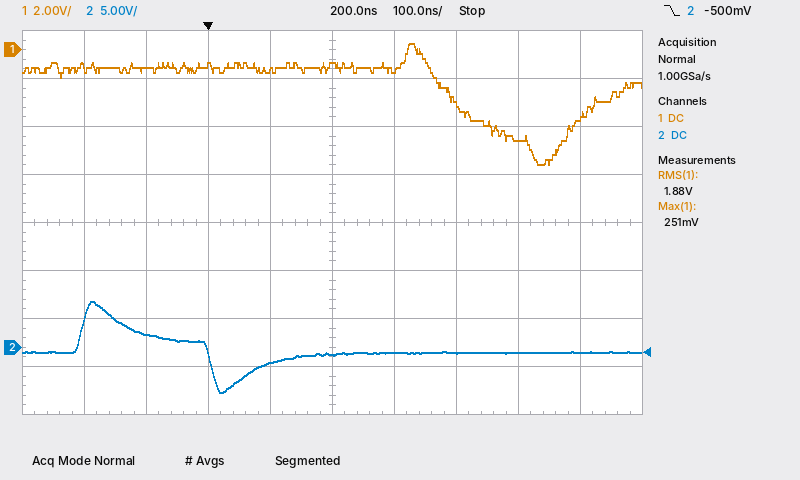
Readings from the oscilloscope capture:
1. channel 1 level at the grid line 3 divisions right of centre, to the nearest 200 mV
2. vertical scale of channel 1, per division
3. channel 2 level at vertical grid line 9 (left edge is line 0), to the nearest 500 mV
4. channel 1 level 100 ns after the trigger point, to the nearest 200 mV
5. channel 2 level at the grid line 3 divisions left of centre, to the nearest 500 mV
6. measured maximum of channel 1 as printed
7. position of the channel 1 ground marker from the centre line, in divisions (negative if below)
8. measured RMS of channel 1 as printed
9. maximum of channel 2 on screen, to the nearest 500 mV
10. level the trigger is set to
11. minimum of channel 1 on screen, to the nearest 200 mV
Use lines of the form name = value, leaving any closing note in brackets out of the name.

channel 1 level at the grid line 3 divisions right of centre, to the nearest 200 mV = -3.8 V
vertical scale of channel 1, per division = 2 V
channel 2 level at vertical grid line 9 (left edge is line 0), to the nearest 500 mV = -500 mV
channel 1 level 100 ns after the trigger point, to the nearest 200 mV = -800 mV
channel 2 level at the grid line 3 divisions left of centre, to the nearest 500 mV = 1.5 V
measured maximum of channel 1 as printed = 251 mV
position of the channel 1 ground marker from the centre line, in divisions = +3.6 div
measured RMS of channel 1 as printed = 1.88 V
maximum of channel 2 on screen, to the nearest 500 mV = 5.0 V
level the trigger is set to = -500 mV
minimum of channel 1 on screen, to the nearest 200 mV = -4.8 V
